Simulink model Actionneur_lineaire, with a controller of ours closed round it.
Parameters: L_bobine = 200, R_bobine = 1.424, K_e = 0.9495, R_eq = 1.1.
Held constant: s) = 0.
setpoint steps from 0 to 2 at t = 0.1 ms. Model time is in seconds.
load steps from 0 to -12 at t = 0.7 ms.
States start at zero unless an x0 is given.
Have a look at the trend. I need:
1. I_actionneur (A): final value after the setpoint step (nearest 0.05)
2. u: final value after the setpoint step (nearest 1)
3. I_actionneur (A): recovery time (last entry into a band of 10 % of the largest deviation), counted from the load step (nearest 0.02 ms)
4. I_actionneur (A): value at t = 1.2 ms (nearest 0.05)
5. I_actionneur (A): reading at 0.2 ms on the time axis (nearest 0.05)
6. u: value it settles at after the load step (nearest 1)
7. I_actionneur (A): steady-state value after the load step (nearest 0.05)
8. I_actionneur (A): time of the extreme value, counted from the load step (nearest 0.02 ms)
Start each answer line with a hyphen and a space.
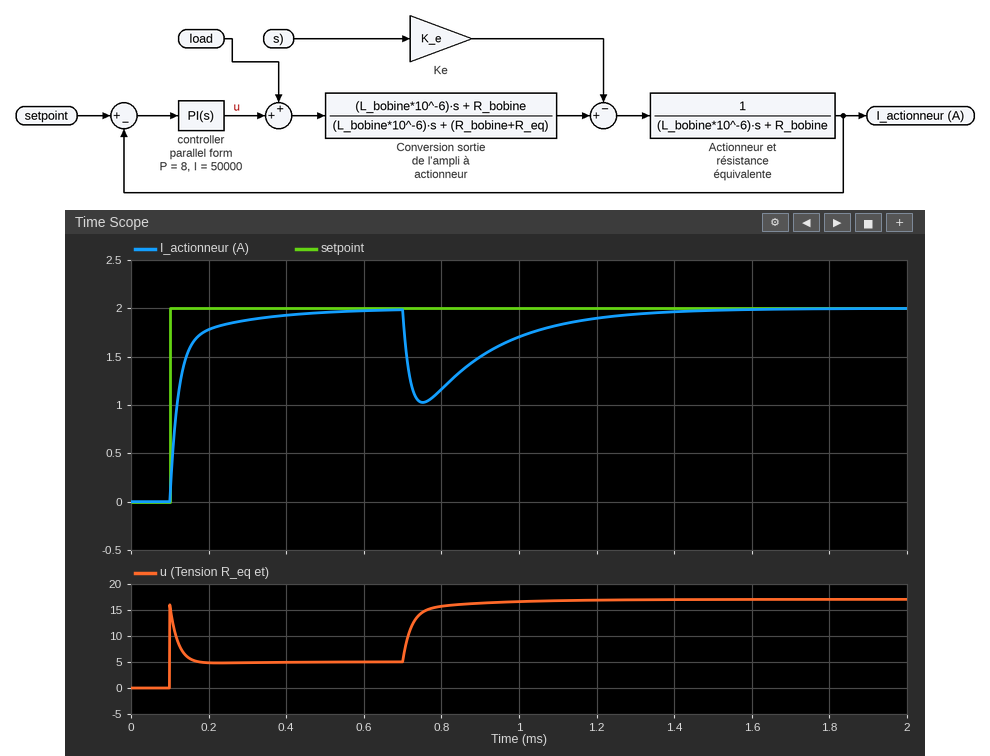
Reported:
- 2.00
- 5
- 0.52 ms
- 1.90
- 1.80
- 17
- 2.00
- 0.06 ms
